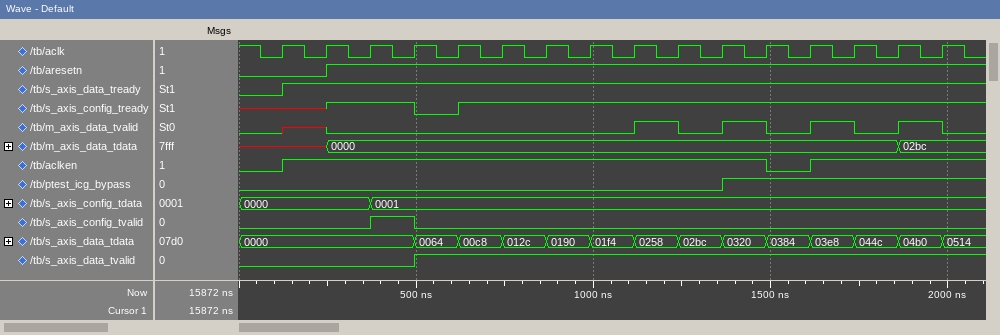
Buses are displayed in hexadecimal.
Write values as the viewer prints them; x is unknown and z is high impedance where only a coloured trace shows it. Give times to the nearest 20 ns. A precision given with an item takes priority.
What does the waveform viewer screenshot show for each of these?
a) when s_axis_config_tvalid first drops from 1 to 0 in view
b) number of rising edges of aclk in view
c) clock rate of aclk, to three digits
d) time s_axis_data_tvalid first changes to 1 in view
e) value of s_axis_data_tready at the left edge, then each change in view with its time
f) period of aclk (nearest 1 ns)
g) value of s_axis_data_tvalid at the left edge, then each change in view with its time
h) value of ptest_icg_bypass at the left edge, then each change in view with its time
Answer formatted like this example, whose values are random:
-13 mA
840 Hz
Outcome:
500 ns
16
8.06 MHz
500 ns
0, 1 at 120 ns
124 ns
0, 1 at 500 ns
0, 1 at 1360 ns
